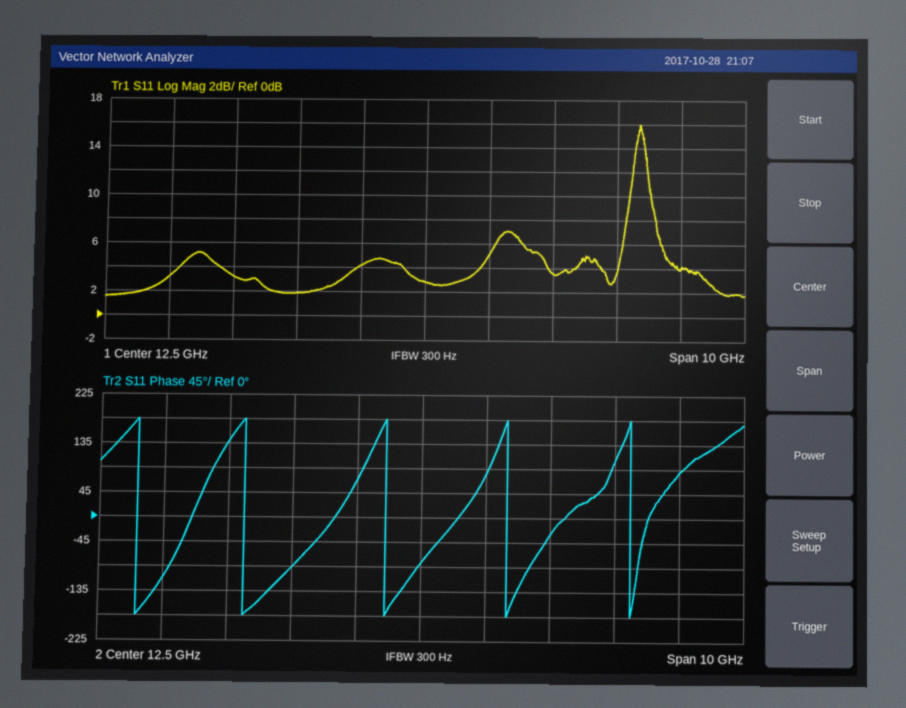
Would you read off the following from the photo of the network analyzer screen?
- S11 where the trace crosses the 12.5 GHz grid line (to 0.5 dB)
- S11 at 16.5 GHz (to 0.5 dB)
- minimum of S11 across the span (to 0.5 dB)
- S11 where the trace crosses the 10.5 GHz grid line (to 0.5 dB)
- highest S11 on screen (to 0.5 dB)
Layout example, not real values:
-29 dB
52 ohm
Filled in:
3.0 dB
4.0 dB
1.5 dB
2.0 dB
16.0 dB
